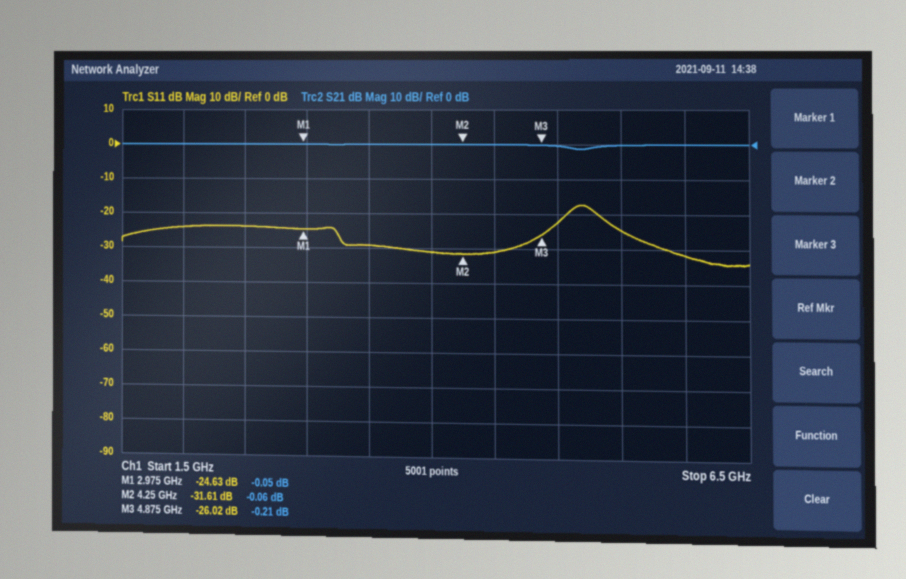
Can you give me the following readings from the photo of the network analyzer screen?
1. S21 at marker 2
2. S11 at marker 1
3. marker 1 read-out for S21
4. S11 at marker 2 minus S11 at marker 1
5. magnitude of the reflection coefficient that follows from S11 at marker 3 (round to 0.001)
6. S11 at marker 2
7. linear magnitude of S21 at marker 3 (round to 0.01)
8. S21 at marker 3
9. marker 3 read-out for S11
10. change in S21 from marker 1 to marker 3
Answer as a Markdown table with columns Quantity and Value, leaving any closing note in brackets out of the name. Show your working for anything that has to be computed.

| Quantity | Value |
|---|---|
| S21 at marker 2 | -0.06 dB |
| S11 at marker 1 | -24.63 dB |
| marker 1 read-out for S21 | -0.05 dB |
| S11 at marker 2 minus S11 at marker 1 | -31.61 − (-24.63) = -6.98 dB |
| magnitude of the reflection coefficient that follows from S11 at marker 3 | 10^(-26.02/20) ≈ 0.050 |
| S11 at marker 2 | -31.61 dB |
| linear magnitude of S21 at marker 3 | 10^(-0.21/20) ≈ 0.98 |
| S21 at marker 3 | -0.21 dB |
| marker 3 read-out for S11 | -26.02 dB |
| change in S21 from marker 1 to marker 3 | -0.21 − (-0.05) = -0.16 dB |
